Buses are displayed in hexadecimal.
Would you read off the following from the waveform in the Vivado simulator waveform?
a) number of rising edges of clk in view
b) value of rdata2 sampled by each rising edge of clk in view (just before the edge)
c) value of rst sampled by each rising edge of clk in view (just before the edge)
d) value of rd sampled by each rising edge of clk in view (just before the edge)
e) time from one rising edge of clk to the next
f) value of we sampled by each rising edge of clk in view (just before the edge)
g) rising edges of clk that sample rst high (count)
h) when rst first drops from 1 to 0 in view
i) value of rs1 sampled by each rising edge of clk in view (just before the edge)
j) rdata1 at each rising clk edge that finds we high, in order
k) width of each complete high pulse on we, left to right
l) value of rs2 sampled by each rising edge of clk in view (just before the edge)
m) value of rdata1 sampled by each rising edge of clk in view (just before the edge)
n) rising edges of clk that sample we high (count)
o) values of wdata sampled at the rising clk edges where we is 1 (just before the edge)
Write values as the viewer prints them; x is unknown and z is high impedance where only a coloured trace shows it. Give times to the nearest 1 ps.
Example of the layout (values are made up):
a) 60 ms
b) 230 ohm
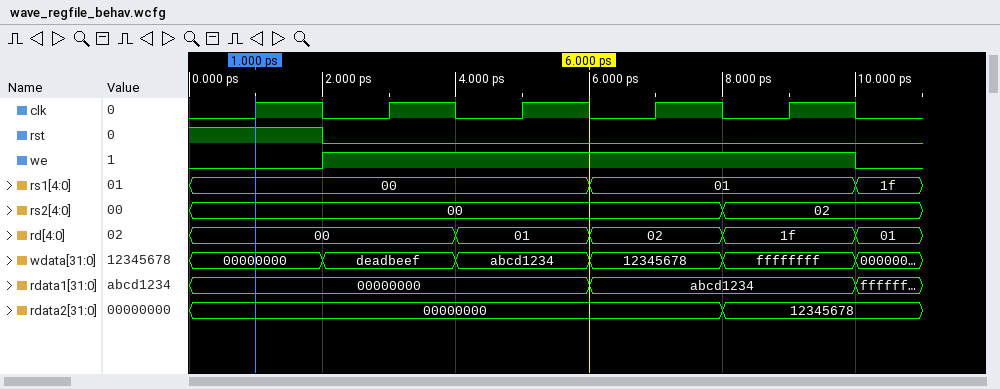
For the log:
a) 5
b) 00000000, 00000000, 00000000, 00000000, 12345678
c) 1 0 0 0 0
d) 00, 00, 01, 02, 1f
e) 2 ps
f) 0 1 1 1 1
g) 1
h) 2 ps
i) 00, 00, 00, 01, 01
j) 00000000, 00000000, abcd1234, abcd1234
k) 8 ps
l) 00, 00, 00, 00, 02
m) 00000000, 00000000, 00000000, abcd1234, abcd1234
n) 4
o) deadbeef, abcd1234, 12345678, ffffffff
